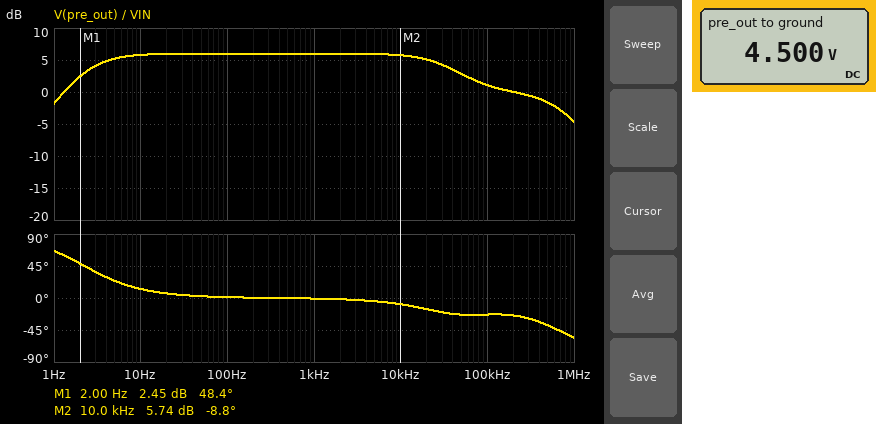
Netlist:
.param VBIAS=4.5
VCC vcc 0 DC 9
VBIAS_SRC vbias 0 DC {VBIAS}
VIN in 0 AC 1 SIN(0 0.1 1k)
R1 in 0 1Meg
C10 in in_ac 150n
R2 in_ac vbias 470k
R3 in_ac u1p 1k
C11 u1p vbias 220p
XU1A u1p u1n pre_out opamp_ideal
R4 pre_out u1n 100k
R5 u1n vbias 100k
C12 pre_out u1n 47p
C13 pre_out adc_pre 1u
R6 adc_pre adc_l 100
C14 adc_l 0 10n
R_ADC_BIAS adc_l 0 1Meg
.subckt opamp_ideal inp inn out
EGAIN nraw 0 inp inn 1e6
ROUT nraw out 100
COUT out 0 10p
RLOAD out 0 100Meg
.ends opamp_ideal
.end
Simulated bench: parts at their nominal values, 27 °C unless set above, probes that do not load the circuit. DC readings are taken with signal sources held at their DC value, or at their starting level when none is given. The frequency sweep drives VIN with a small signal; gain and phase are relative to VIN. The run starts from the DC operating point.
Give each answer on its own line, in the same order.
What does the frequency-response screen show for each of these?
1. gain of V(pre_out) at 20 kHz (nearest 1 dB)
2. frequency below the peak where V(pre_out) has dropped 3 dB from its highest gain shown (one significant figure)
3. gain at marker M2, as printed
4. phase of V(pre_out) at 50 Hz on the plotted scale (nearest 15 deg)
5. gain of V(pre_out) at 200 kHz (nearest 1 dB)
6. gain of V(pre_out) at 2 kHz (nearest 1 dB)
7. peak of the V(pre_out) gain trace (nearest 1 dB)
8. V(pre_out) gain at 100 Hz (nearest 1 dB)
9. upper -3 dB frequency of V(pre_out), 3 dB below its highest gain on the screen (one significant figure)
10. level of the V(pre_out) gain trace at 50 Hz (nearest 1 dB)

5 dB
2 Hz
5.74 dB
0 deg
0 dB
6 dB
6 dB
6 dB
50 kHz
6 dB
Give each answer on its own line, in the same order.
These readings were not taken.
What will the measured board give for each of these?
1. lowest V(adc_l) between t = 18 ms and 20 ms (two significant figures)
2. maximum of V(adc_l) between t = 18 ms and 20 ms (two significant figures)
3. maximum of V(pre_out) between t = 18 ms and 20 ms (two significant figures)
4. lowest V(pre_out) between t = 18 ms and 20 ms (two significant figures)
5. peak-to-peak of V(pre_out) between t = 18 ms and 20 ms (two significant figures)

-200 mV
200 mV
4.7 V
4.3 V
400 mV
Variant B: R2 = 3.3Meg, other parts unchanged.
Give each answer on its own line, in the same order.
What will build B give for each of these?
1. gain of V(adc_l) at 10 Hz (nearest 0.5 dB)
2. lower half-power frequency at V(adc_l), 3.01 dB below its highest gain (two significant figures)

6.0 dB
380 mHz
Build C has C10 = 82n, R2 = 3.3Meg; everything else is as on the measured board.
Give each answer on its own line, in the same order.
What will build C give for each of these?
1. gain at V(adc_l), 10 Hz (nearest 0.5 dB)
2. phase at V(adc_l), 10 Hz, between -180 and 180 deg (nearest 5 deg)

6.0 dB
5 deg
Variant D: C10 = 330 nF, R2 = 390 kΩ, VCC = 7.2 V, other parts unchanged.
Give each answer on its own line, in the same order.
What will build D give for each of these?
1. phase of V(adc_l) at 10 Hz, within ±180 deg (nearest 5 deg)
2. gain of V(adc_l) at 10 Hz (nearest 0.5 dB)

10 deg
6.0 dB
